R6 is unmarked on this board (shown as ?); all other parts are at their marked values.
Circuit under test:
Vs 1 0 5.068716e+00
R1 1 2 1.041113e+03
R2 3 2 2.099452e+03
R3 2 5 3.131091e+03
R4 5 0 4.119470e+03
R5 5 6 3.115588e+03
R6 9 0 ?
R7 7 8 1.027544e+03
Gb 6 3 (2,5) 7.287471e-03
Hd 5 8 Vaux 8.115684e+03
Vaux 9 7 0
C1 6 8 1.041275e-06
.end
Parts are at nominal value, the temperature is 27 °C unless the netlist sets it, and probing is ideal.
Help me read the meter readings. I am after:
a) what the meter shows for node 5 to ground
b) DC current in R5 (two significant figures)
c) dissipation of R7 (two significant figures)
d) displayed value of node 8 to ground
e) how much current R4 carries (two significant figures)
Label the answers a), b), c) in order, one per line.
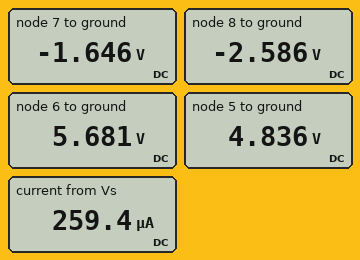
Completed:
a) 4.836 V
b) 270 µA
c) 860 µW
d) -2.586 V
e) 1.2 mA
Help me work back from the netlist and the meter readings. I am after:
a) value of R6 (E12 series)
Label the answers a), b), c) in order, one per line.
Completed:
a) 1.8 kΩ
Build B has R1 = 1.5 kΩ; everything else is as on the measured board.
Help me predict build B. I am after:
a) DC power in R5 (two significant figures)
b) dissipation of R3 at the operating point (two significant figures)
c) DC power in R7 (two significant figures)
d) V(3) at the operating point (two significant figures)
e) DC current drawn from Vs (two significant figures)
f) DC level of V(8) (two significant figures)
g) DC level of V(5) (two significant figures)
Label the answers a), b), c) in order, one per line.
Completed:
a) 220 µW
b) 420 nW
c) 820 µW
d) 4.1 V
e) 250 µA
f) -2.5 V
g) 4.7 V
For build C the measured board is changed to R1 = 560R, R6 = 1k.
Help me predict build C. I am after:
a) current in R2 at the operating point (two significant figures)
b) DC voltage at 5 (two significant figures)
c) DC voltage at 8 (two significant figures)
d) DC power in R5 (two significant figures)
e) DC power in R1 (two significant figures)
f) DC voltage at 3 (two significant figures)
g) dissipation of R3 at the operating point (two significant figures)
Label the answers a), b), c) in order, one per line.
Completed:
a) 400 µA
b) 4.9 V
c) -1.6 V
d) 510 µW
e) 83 µW
f) 4.0 V
g) 980 nW
